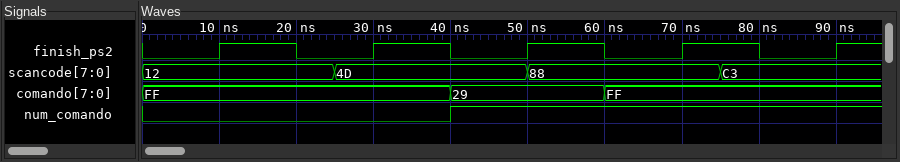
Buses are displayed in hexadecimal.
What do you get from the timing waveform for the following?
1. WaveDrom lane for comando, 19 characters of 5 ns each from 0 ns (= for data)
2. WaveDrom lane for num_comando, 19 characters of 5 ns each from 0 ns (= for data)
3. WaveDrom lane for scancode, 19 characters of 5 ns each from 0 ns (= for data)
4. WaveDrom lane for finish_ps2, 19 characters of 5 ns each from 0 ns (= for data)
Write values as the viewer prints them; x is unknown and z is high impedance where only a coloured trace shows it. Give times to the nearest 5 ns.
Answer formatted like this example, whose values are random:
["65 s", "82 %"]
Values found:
["{name: 'comando', wave: '=.......=...=......', data: 'FF 29 FF'}", "{name: 'num_comando', wave: '0.......1..........'}", "{name: 'scancode', wave: '=....=....=....=...', data: '12 4D 88 C3'}", "{name: 'finish_ps2', wave: '0.1.0.1.0.1.0.1.0.1'}"]
